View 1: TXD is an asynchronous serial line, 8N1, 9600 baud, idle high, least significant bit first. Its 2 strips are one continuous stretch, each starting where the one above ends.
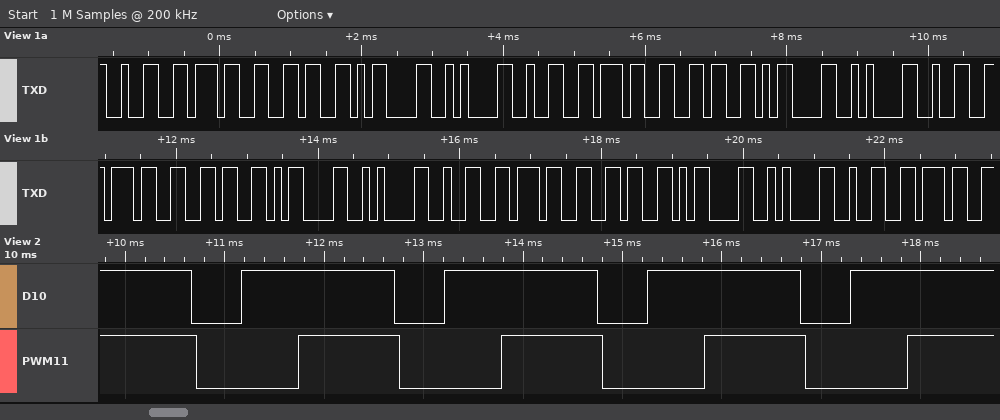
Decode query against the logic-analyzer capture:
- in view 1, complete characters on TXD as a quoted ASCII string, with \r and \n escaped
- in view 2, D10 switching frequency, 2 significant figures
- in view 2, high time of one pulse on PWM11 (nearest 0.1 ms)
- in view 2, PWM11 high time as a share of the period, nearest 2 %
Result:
"276\r\n276\r\n276\r\n276\r\n27"
490 Hz
1.0 ms
50 %
